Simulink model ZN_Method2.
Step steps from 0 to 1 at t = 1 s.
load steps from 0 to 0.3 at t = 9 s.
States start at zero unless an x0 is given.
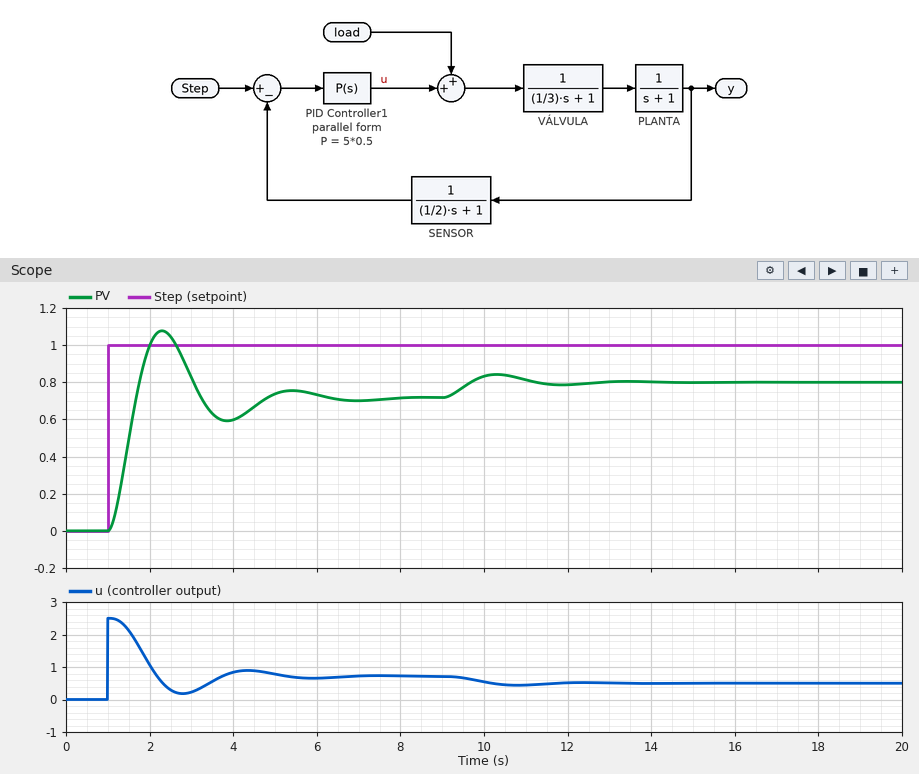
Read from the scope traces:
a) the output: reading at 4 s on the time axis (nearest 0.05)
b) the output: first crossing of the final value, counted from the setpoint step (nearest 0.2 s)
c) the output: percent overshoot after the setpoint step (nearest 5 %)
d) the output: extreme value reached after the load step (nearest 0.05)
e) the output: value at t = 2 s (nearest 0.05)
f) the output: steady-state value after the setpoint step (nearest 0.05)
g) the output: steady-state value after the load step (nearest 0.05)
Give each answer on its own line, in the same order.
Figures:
0.60
0.6 s
50 %
0.85
1.00
0.70
0.80
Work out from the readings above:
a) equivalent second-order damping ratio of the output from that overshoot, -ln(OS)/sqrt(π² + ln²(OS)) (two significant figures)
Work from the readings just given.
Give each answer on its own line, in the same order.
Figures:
0.22
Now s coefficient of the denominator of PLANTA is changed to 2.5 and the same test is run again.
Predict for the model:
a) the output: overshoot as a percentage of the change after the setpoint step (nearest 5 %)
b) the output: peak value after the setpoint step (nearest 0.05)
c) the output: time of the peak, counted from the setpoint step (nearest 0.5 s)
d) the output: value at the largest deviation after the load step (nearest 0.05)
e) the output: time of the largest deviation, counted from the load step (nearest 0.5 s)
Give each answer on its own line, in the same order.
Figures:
20 %
0.85
2.0 s
0.80
2.0 s
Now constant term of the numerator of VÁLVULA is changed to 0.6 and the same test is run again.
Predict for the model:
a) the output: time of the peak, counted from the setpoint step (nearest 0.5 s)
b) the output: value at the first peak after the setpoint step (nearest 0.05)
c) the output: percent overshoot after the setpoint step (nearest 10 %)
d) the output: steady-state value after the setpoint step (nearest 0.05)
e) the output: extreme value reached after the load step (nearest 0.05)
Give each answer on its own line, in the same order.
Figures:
1.5 s
0.75
30 %
0.60
0.70
